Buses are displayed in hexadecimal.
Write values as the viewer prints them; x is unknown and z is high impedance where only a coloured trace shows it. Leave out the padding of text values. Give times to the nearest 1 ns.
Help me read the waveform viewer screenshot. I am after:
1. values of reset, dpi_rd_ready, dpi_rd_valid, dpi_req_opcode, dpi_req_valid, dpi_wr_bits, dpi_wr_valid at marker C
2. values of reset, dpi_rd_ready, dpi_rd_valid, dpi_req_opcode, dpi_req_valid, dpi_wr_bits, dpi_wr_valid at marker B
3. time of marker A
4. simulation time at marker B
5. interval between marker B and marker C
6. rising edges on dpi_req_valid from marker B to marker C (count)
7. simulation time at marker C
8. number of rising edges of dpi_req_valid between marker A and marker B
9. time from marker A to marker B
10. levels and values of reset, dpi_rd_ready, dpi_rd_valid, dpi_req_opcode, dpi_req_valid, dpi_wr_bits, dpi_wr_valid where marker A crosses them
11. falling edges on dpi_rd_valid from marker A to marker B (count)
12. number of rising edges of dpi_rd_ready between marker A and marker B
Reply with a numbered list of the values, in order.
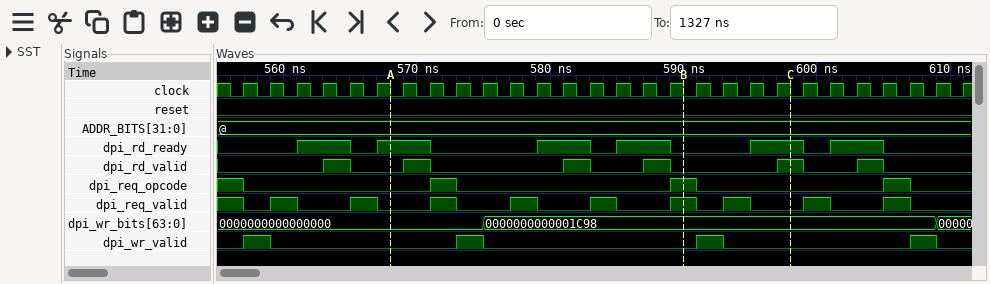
1. reset=0, dpi_rd_ready=1, dpi_rd_valid=1, dpi_req_opcode=0, dpi_req_valid=0, dpi_wr_bits=0000000000001C98, dpi_wr_valid=0
2. reset=0, dpi_rd_ready=0, dpi_rd_valid=0, dpi_req_opcode=1, dpi_req_valid=1, dpi_wr_bits=0000000000001C98, dpi_wr_valid=0
3. 568 ns
4. 590 ns
5. 8 ns
6. 1
7. 598 ns
8. 4
9. 22 ns
10. reset=0, dpi_rd_ready=1, dpi_rd_valid=0, dpi_req_opcode=0, dpi_req_valid=0, dpi_wr_bits=0000000000000000, dpi_wr_valid=0
11. 3
12. 2
